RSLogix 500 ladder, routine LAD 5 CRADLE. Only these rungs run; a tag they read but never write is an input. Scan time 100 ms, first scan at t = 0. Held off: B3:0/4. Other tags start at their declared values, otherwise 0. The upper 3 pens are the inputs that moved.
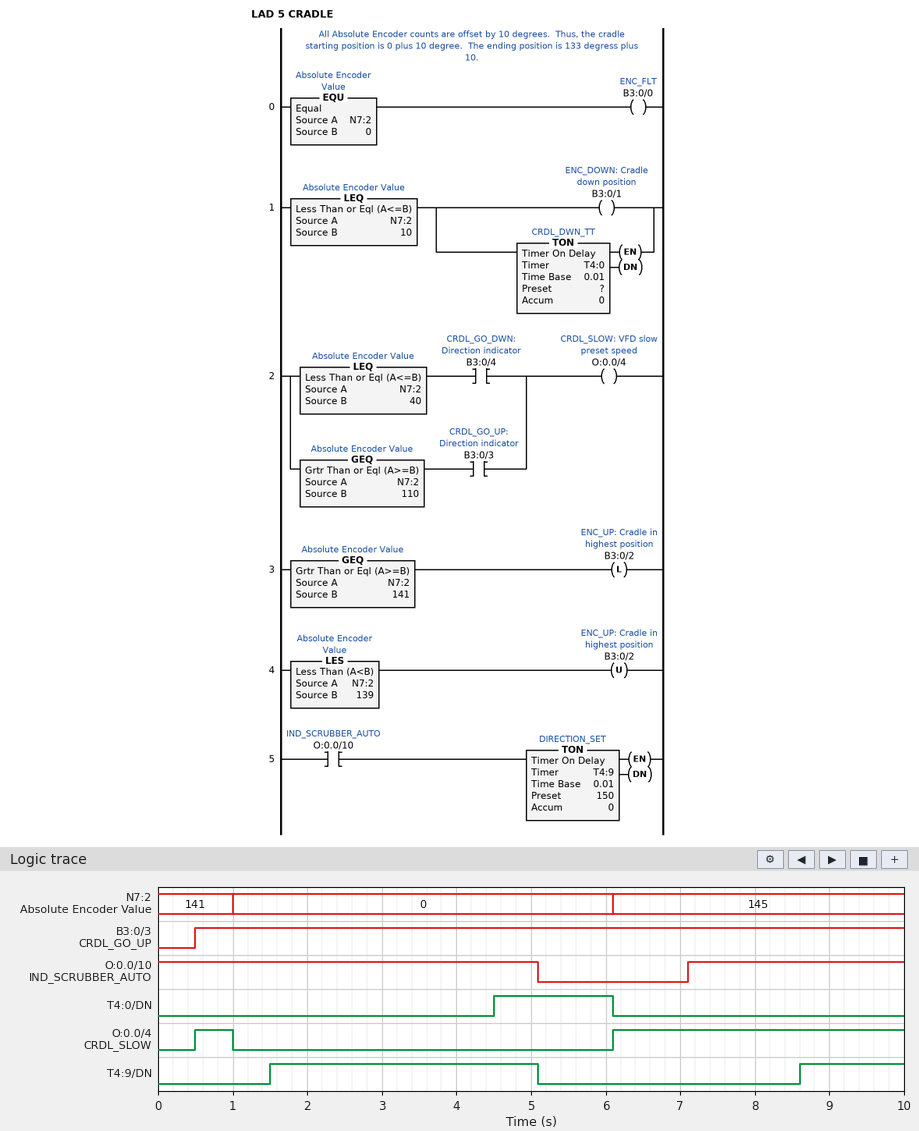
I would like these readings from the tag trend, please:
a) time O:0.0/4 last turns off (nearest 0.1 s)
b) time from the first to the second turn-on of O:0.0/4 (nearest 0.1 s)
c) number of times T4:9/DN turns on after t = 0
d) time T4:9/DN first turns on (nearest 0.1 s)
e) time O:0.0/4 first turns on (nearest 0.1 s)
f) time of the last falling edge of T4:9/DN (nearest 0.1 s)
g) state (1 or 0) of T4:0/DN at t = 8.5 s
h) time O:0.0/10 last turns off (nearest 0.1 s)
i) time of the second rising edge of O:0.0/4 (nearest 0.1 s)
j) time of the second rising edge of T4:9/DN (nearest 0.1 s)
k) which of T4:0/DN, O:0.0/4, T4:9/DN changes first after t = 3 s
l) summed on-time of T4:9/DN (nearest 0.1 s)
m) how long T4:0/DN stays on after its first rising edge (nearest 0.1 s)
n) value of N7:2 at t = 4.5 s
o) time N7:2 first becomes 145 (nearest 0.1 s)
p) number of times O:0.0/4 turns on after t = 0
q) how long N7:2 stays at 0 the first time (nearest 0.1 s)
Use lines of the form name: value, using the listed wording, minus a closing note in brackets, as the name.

time O:0.0/4 last turns off: 1.0 s
time from the first to the second turn-on of O:0.0/4: 5.6 s
number of times T4:9/DN turns on after t = 0: 2
time T4:9/DN first turns on: 1.5 s
time O:0.0/4 first turns on: 0.5 s
time of the last falling edge of T4:9/DN: 5.1 s
state (1 or 0) of T4:0/DN at t = 8.5 s: 0
time O:0.0/10 last turns off: 5.1 s
time of the second rising edge of O:0.0/4: 6.1 s
time of the second rising edge of T4:9/DN: 8.6 s
which of T4:0/DN, O:0.0/4, T4:9/DN changes first after t = 3 s: T4:0/DN
summed on-time of T4:9/DN: 5.0 s
how long T4:0/DN stays on after its first rising edge: 1.6 s
value of N7:2 at t = 4.5 s: 0
time N7:2 first becomes 145: 6.1 s
number of times O:0.0/4 turns on after t = 0: 2
how long N7:2 stays at 0 the first time: 5.1 s
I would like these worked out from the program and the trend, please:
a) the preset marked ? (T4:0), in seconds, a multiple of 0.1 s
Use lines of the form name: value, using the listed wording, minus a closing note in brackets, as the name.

the preset marked ? (T4:0), in seconds, a multiple of 0.1 s: 3.5 s
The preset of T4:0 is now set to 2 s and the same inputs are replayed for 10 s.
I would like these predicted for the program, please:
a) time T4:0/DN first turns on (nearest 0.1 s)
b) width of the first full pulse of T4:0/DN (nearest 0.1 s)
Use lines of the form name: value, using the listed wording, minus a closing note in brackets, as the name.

time T4:0/DN first turns on: 3.0 s
width of the first full pulse of T4:0/DN: 3.1 s
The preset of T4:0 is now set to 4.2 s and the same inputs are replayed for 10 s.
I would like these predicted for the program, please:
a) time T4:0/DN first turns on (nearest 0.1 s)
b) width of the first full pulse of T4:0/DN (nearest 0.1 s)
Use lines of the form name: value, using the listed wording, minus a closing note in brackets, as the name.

time T4:0/DN first turns on: 5.2 s
width of the first full pulse of T4:0/DN: 0.9 s
